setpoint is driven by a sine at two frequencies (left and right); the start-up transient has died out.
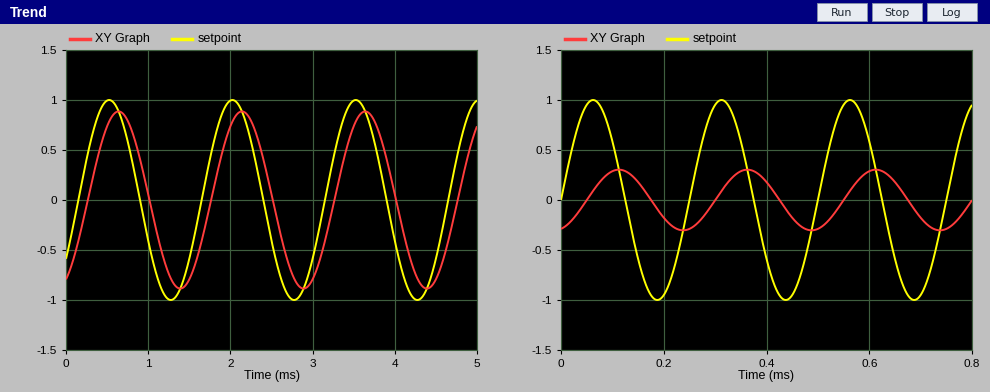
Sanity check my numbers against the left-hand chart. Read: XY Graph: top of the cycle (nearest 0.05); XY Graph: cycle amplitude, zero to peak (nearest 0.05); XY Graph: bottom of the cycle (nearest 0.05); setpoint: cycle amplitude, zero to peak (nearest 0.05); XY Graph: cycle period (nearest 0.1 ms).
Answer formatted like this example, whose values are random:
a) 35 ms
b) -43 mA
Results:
a) 0.90
b) 0.90
c) -0.90
d) 1.00
e) 1.5 ms
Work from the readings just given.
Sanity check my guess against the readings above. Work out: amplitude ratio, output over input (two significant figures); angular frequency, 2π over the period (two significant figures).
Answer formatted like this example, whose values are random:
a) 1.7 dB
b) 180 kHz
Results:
a) 0.90
b) 4.2 rad/ms
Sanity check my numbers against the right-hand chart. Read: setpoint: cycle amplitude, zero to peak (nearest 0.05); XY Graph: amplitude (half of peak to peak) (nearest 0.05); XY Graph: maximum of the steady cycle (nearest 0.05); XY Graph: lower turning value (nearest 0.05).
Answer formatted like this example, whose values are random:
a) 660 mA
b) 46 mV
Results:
a) 1.00
b) 0.30
c) 0.30
d) -0.30
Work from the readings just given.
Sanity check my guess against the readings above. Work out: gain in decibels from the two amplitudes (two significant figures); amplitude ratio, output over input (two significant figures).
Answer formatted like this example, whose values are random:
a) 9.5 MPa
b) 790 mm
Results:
a) -10 dB
b) 0.30
